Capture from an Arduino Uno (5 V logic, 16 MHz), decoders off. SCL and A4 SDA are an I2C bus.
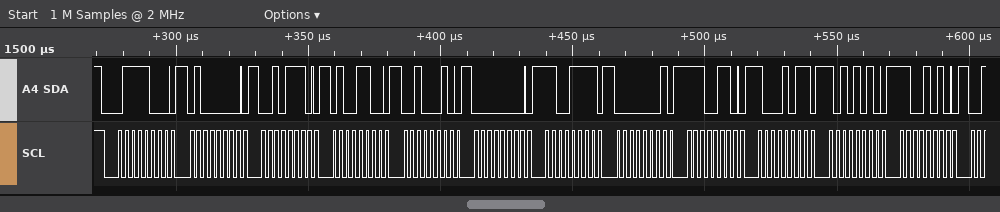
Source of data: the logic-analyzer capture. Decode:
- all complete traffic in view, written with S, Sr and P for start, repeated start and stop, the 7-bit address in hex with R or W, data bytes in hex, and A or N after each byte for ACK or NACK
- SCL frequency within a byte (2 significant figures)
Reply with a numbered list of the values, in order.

1. S 3CW A 40 A 2E A 4C A 22 A 00 A CF A 01 A E6 A 8B A AA A CA A
2. 400 kHz
